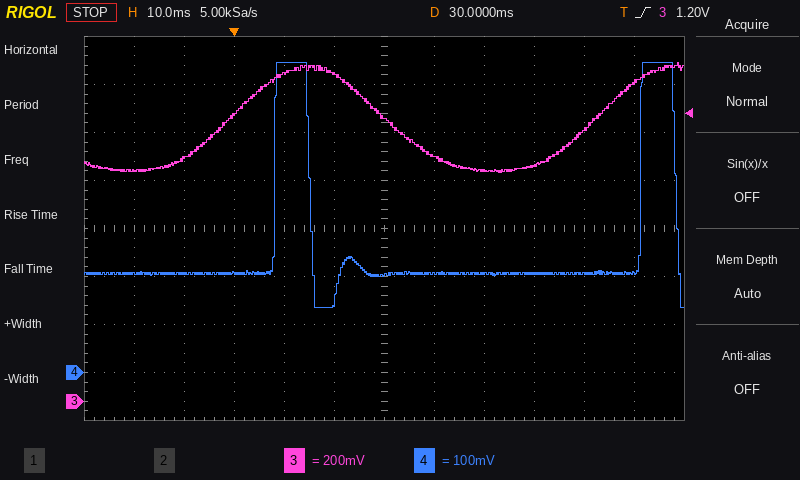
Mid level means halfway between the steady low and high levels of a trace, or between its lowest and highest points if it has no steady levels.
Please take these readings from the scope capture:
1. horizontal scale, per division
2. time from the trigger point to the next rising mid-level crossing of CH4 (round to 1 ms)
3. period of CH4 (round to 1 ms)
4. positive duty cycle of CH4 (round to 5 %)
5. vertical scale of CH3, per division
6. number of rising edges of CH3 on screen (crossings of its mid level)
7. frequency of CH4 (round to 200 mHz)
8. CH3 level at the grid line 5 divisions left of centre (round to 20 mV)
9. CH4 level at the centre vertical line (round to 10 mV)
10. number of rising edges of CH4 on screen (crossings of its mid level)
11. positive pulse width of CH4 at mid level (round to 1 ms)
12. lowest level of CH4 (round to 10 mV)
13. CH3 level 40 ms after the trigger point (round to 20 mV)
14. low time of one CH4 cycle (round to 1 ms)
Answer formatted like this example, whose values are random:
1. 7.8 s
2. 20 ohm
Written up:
1. 10 ms
2. 8 ms
3. 73 ms
4. 10 %
5. 200 mV
6. 2
7. 13.6 Hz
8. 960 mV
9. 200 mV
10. 2
11. 7 ms
12. 140 mV
13. 1.02 V
14. 66 ms
